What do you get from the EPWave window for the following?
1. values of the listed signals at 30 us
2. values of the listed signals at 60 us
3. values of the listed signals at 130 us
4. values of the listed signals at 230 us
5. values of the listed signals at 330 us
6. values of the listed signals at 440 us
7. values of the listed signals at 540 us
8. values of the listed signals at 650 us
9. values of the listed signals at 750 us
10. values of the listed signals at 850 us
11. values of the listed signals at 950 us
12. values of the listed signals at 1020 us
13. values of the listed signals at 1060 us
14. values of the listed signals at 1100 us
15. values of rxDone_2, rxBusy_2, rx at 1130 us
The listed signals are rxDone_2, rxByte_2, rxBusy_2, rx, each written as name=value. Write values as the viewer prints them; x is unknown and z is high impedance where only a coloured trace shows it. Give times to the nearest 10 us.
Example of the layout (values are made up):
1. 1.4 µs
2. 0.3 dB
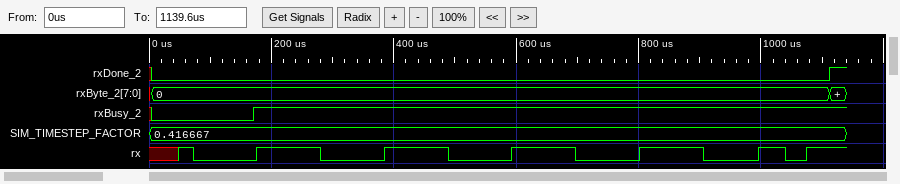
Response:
1. rxDone_2=0, rxByte_2=0, rxBusy_2=0, rx=x
2. rxDone_2=0, rxByte_2=0, rxBusy_2=0, rx=1
3. rxDone_2=0, rxByte_2=0, rxBusy_2=0, rx=0
4. rxDone_2=0, rxByte_2=0, rxBusy_2=1, rx=1
5. rxDone_2=0, rxByte_2=0, rxBusy_2=1, rx=0
6. rxDone_2=0, rxByte_2=0, rxBusy_2=1, rx=1
7. rxDone_2=0, rxByte_2=0, rxBusy_2=1, rx=0
8. rxDone_2=0, rxByte_2=0, rxBusy_2=1, rx=1
9. rxDone_2=0, rxByte_2=0, rxBusy_2=1, rx=0
10. rxDone_2=0, rxByte_2=0, rxBusy_2=1, rx=1
11. rxDone_2=0, rxByte_2=0, rxBusy_2=1, rx=0
12. rxDone_2=0, rxByte_2=0, rxBusy_2=1, rx=1
13. rxDone_2=0, rxByte_2=0, rxBusy_2=1, rx=0
14. rxDone_2=0, rxByte_2=0, rxBusy_2=1, rx=1
15. rxDone_2=1, rxBusy_2=1, rx=1
